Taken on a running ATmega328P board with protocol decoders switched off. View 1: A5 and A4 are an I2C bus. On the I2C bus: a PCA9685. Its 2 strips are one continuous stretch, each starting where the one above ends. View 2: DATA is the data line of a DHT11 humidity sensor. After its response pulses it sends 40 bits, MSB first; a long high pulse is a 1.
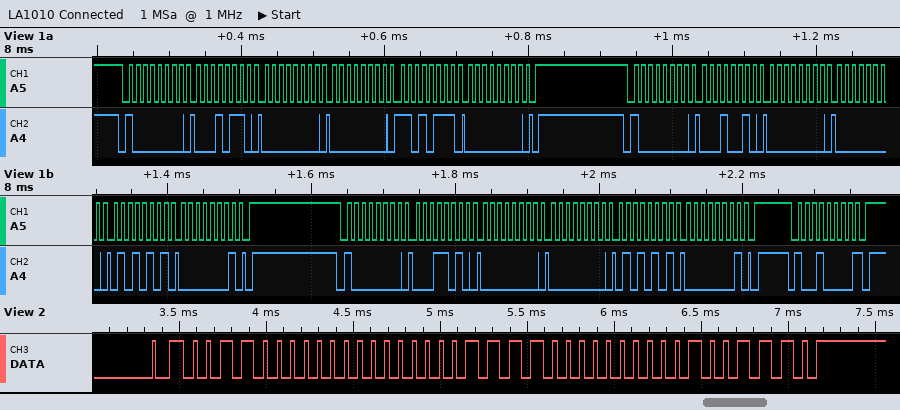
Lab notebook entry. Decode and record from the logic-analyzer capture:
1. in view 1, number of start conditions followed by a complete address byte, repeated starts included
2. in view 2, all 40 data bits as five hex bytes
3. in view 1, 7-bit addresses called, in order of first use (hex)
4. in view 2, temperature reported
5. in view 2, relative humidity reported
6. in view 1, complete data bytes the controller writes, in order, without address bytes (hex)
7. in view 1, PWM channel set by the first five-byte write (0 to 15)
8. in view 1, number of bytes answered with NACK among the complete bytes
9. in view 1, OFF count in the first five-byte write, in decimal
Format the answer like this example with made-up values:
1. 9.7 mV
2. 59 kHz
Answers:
1. 4
2. 30 00 1E 00 4E
3. 0x40 0x48
4. 30.0 °C
5. 48 %
6. 16 00 00 D7 00 12 00 00 55 01 1A 00 00 55 01
7. 4
8. 1
9. 215
